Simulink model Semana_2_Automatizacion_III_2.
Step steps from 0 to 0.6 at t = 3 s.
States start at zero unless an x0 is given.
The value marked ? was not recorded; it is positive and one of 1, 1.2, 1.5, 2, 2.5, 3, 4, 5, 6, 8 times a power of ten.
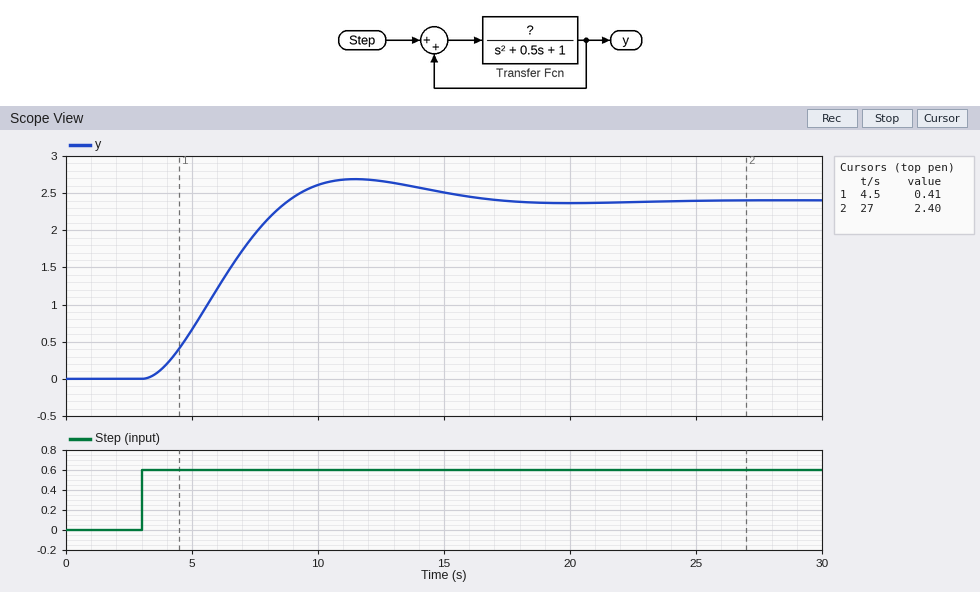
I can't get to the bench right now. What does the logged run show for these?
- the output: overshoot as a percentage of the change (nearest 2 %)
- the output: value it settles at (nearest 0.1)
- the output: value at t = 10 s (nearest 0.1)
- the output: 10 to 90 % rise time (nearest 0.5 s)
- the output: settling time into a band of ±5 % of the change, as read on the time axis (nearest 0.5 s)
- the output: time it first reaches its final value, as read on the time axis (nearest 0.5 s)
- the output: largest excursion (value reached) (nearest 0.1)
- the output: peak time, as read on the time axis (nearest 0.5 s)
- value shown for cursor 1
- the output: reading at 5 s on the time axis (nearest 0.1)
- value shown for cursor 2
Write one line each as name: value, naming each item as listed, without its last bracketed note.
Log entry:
the output: overshoot as a percentage of the change: 12 %
the output: value it settles at: 2.4
the output: value at t = 10 s: 2.6
the output: 10 to 90 % rise time: 4.0 s
the output: settling time into a band of ±5 % of the change, as read on the time axis: 15.0 s
the output: time it first reaches its final value, as read on the time axis: 9.0 s
the output: largest excursion (value reached): 2.7
the output: peak time, as read on the time axis: 11.5 s
value shown for cursor 1: 0.41
the output: reading at 5 s on the time axis: 0.7
value shown for cursor 2: 2.40
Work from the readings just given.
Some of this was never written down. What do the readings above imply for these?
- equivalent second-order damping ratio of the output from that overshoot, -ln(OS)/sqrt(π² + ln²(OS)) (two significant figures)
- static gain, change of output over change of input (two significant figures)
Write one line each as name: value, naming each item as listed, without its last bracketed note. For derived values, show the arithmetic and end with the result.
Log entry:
equivalent second-order damping ratio of the output from that overshoot, -ln(OS)/sqrt(π² + ln²(OS)): ln(0.12) = -2.120; 2.120 / sqrt(9.870 + 4.496) = 0.56
static gain, change of output over change of input: (2.4 - 0) / (0.6 - 0) = 4.0
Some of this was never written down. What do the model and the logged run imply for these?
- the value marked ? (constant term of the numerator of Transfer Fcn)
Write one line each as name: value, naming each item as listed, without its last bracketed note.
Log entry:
the value marked ?: 0.8
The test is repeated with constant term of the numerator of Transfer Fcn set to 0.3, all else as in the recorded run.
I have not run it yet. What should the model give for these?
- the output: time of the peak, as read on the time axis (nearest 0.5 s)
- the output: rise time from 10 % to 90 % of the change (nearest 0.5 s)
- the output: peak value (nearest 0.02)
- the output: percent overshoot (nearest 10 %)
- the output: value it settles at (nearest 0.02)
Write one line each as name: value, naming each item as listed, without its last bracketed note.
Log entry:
the output: time of the peak, as read on the time axis: 7.0 s
the output: rise time from 10 % to 90 % of the change: 1.5 s
the output: peak value: 0.36
the output: percent overshoot: 40 %
the output: value it settles at: 0.26
